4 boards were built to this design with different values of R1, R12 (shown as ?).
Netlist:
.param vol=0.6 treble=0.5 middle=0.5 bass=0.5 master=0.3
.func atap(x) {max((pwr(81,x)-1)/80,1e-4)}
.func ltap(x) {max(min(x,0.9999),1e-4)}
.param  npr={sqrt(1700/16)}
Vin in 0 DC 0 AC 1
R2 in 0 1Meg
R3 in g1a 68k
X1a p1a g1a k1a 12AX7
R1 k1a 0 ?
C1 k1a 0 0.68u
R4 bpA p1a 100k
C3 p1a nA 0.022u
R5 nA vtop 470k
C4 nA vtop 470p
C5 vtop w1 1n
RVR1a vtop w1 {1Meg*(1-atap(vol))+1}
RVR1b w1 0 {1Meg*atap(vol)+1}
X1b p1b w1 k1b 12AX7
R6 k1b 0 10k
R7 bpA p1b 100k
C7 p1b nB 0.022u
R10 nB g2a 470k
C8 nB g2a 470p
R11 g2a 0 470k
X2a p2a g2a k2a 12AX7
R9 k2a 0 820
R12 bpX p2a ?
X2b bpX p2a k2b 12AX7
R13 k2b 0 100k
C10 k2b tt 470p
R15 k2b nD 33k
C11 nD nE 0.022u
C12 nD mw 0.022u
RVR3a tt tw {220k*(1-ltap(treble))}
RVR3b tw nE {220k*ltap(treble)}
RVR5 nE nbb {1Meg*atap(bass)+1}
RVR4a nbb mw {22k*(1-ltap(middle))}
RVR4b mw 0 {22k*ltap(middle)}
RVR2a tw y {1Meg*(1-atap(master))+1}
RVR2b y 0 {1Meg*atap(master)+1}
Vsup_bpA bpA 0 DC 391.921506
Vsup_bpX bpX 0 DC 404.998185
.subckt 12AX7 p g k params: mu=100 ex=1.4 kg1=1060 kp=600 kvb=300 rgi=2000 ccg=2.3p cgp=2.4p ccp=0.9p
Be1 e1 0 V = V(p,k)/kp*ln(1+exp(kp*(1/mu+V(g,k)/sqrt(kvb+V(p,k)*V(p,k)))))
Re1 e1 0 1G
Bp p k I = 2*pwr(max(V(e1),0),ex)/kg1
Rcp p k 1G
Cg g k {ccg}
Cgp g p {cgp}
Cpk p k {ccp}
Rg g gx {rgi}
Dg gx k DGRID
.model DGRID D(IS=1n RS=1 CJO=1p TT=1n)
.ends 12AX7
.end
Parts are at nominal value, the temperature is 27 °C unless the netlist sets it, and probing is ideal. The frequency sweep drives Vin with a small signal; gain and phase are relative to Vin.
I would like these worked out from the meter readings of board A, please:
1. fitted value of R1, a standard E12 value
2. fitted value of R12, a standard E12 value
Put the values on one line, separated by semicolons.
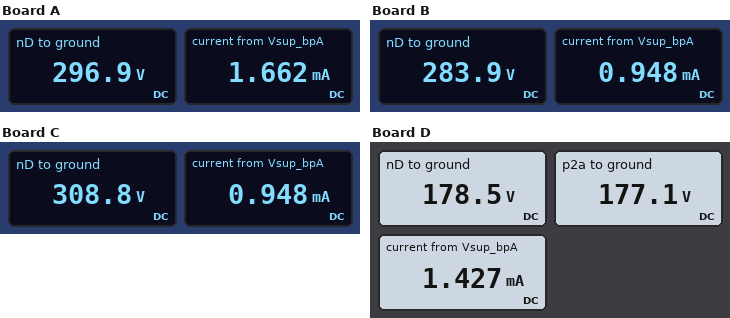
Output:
1.5 kΩ; 47 kΩ
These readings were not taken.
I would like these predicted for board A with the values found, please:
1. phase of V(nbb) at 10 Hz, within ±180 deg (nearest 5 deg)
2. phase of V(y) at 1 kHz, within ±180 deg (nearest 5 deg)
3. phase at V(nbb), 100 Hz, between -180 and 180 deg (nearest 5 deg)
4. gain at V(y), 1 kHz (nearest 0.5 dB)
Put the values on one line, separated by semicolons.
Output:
-40 deg; -105 deg; -110 deg; 27.0 dB
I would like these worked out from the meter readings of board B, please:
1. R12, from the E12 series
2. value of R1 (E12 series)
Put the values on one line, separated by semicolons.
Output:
56 kΩ; 5.6 kΩ
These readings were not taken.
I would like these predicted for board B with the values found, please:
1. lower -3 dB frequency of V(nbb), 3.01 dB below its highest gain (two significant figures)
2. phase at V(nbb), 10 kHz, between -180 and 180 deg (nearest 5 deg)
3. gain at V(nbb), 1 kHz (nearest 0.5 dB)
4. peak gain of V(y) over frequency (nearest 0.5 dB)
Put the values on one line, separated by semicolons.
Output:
2.4 kHz; 155 deg; 53.0 dB; 40.0 dB
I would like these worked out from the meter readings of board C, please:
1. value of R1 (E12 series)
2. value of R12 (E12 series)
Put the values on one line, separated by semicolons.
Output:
5.6 kΩ; 39 kΩ
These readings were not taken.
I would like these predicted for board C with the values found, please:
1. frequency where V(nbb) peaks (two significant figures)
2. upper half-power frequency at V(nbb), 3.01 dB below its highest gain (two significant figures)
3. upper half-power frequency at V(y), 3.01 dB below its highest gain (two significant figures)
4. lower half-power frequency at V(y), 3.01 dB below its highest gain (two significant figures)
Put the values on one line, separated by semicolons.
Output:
7.7 kHz; 23 kHz; 24 kHz; 2.9 kHz
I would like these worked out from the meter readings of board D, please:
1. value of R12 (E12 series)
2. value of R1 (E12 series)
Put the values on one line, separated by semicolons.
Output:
180 kΩ; 2.2 kΩ
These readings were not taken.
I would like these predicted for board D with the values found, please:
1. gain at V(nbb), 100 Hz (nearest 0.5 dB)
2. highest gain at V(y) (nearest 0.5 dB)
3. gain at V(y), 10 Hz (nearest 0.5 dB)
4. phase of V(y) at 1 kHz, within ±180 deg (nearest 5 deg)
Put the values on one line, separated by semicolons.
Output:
42.5 dB; 46.5 dB; 6.0 dB; -110 deg
